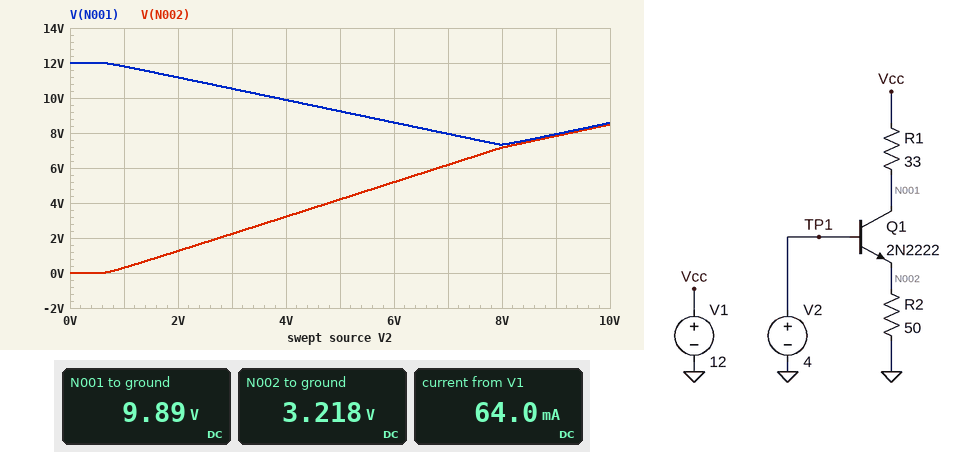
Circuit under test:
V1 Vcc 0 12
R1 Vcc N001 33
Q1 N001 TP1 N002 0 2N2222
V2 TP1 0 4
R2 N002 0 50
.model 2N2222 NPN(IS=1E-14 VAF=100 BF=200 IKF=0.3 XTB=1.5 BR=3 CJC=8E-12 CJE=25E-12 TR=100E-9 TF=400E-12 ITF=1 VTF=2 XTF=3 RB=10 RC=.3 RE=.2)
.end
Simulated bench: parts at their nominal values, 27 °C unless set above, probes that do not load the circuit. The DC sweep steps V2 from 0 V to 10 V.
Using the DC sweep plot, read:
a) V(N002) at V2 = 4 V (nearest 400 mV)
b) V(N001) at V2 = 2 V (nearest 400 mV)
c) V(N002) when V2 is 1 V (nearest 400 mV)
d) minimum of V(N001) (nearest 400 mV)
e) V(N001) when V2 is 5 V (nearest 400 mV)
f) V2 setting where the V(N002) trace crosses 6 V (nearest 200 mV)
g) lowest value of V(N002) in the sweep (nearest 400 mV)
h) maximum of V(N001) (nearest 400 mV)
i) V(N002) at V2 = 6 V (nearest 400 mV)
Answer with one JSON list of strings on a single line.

["3.2 V", "11.2 V", "400 mV", "7.2 V", "9.2 V", "6.8 V", "0 V", "12.0 V", "5.2 V"]
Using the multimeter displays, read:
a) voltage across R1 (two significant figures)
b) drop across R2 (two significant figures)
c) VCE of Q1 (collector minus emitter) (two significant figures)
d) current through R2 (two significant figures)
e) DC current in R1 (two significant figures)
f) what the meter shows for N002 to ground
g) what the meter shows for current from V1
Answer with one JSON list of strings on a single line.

["2.1 V", "3.2 V", "6.7 V", "64 mA", "64 mA", "3.218 V", "64.0 mA"]
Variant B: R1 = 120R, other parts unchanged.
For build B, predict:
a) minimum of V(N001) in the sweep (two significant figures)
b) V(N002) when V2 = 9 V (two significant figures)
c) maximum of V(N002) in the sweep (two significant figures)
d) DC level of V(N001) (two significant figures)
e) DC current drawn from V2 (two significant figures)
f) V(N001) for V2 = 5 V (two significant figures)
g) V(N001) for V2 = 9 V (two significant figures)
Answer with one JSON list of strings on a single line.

["3.7 V", "7.1 V", "7.9 V", "4.3 V", "390 µA", "4.1 V", "7.2 V"]
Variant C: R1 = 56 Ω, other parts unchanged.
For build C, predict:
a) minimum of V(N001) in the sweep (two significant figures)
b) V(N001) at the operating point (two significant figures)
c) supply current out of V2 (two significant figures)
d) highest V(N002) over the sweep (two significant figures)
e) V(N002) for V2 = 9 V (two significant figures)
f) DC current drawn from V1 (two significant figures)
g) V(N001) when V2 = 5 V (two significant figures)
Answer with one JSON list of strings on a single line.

["5.8 V", "8.4 V", "370 µA", "8.2 V", "7.5 V", "64 mA", "7.3 V"]
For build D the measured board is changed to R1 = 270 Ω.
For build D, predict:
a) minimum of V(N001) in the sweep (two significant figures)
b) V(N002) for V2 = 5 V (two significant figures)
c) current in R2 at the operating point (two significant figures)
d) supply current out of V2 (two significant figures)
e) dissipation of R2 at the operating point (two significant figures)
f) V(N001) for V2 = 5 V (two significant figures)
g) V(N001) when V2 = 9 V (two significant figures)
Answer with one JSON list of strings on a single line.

["2.0 V", "3.7 V", "59 mA", "26 mA", "170 mW", "3.8 V", "7.0 V"]
